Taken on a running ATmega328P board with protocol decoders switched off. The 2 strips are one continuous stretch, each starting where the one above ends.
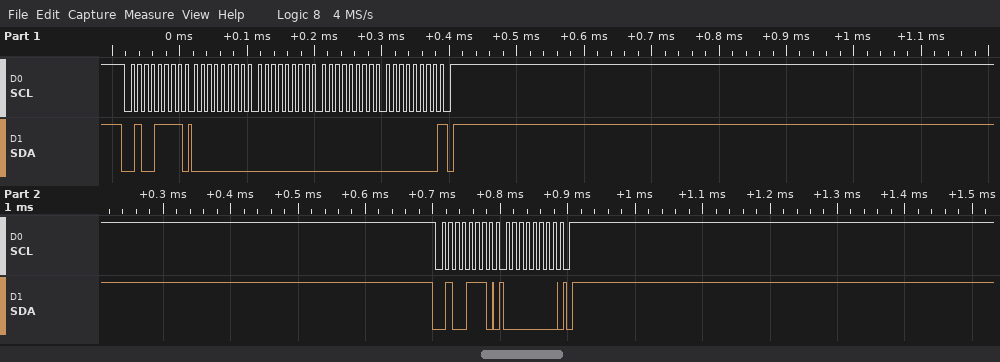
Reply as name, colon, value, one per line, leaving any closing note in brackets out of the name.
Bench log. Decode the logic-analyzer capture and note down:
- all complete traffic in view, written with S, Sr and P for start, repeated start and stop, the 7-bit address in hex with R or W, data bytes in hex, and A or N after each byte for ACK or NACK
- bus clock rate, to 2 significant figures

all complete traffic in view, written with S, Sr and P for start, repeated start and stop, the 7-bit address in hex with R or W, data bytes in hex, and A or N after each byte for ACK or NACK: S 27R A 00 A 00 A 00 A 00 N P S 27W A 00 A P
bus clock rate, to 2 significant figures: 100 kHz
